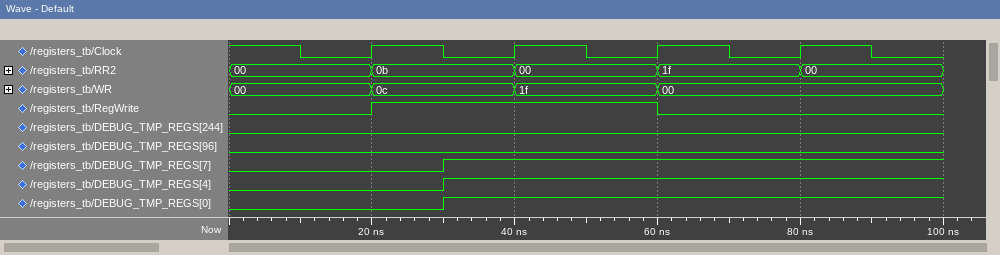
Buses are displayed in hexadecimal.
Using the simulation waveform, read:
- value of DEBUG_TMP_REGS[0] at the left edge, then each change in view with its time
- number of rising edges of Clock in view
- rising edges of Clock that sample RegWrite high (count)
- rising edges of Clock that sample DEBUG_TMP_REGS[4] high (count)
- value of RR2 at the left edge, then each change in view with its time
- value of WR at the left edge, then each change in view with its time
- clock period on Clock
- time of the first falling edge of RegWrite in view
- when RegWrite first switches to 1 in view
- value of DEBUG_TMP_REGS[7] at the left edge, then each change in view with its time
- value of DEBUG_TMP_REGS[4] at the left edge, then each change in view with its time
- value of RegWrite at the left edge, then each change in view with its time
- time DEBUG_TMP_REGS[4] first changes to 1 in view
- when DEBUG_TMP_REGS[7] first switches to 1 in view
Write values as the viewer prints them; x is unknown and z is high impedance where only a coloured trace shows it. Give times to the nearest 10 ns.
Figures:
0, 1 at 30 ns
4
2
3
00, 0b at 20 ns, 00 at 40 ns, 1f at 60 ns, 00 at 80 ns
00, 0c at 20 ns, 1f at 40 ns, 00 at 60 ns
20 ns
60 ns
20 ns
0, 1 at 30 ns
0, 1 at 30 ns
0, 1 at 20 ns, 0 at 60 ns
30 ns
30 ns
